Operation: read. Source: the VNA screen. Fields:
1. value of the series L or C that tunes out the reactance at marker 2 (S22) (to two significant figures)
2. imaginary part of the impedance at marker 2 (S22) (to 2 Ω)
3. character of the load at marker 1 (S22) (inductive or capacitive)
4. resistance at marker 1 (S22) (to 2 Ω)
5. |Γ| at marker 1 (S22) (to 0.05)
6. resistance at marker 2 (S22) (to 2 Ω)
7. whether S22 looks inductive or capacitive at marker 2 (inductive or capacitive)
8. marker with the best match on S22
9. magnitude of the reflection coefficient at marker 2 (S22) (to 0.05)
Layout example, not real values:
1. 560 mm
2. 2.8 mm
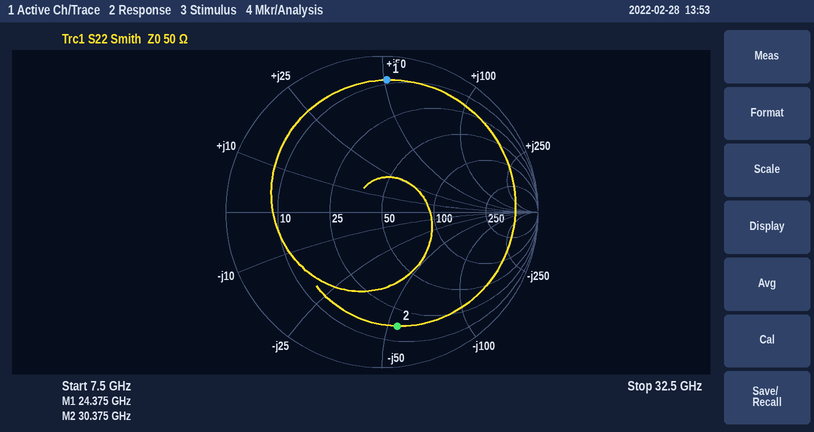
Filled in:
1. 280 pH
2. -54 Ω
3. inductive
4. 8 Ω
5. 0.85
6. 16 Ω
7. capacitive
8. marker 2
9. 0.75
